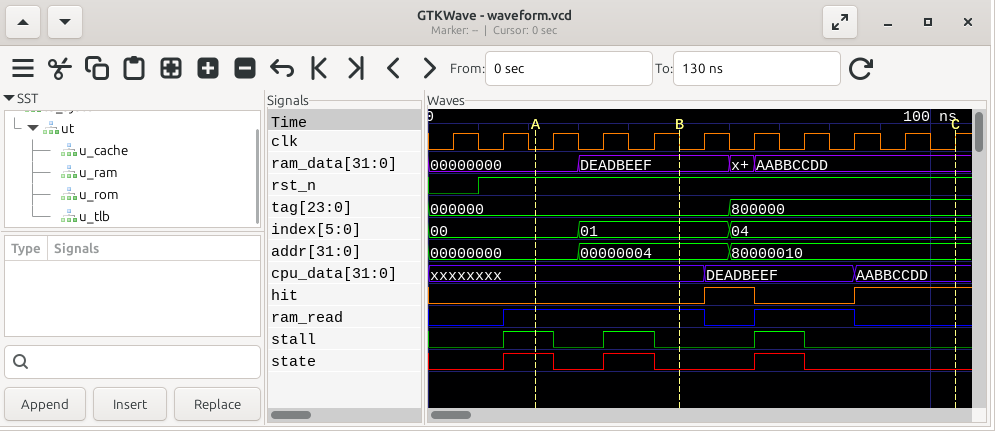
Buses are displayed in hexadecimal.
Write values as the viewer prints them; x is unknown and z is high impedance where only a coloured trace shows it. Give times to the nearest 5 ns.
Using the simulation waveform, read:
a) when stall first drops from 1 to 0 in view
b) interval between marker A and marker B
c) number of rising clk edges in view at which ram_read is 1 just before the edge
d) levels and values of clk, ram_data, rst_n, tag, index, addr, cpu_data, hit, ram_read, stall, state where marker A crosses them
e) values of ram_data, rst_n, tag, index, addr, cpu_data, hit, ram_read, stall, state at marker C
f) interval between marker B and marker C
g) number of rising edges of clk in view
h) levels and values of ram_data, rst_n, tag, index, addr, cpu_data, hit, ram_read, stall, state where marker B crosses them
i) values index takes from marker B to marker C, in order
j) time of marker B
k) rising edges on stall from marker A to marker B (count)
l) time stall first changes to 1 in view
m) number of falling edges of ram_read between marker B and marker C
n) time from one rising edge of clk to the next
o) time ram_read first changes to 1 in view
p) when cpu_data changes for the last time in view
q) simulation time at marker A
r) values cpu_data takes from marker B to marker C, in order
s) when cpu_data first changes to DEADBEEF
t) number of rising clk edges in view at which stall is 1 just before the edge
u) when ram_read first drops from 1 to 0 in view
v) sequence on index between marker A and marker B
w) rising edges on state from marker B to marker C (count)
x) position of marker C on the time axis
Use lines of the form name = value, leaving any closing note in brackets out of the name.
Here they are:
when stall first drops from 1 to 0 in view = 25 ns
interval between marker A and marker B = 30 ns
number of rising clk edges in view at which ram_read is 1 just before the edge = 6
levels and values of clk, ram_data, rst_n, tag, index, addr, cpu_data, hit, ram_read, stall, state where marker A crosses them = clk=0, ram_data=00000000, rst_n=1, tag=000000, index=00, addr=00000000, cpu_data=xxxxxxxx, hit=0, ram_read=1, stall=1, state=1
values of ram_data, rst_n, tag, index, addr, cpu_data, hit, ram_read, stall, state at marker C = ram_data=AABBCCDD, rst_n=1, tag=800000, index=04, addr=80000010, cpu_data=AABBCCDD, hit=1, ram_read=0, stall=0, state=0
interval between marker B and marker C = 55 ns
number of rising edges of clk in view = 11
levels and values of ram_data, rst_n, tag, index, addr, cpu_data, hit, ram_read, stall, state where marker B crosses them = ram_data=DEADBEEF, rst_n=1, tag=000000, index=01, addr=00000004, cpu_data=xxxxxxxx, hit=0, ram_read=1, stall=0, state=0
values index takes from marker B to marker C, in order = 01, 04
time of marker B = 50 ns
rising edges on stall from marker A to marker B = 1
time stall first changes to 1 in view = 15 ns
number of falling edges of ram_read between marker B and marker C = 2
time from one rising edge of clk to the next = 10 ns
time ram_read first changes to 1 in view = 15 ns
when cpu_data changes for the last time in view = 85 ns
simulation time at marker A = 20 ns
values cpu_data takes from marker B to marker C, in order = xxxxxxxx, DEADBEEF, AABBCCDD
when cpu_data first changes to DEADBEEF = 55 ns
number of rising clk edges in view at which stall is 1 just before the edge = 3
when ram_read first drops from 1 to 0 in view = 55 ns
sequence on index between marker A and marker B = 00, 01
rising edges on state from marker B to marker C = 1
position of marker C on the time axis = 105 ns
